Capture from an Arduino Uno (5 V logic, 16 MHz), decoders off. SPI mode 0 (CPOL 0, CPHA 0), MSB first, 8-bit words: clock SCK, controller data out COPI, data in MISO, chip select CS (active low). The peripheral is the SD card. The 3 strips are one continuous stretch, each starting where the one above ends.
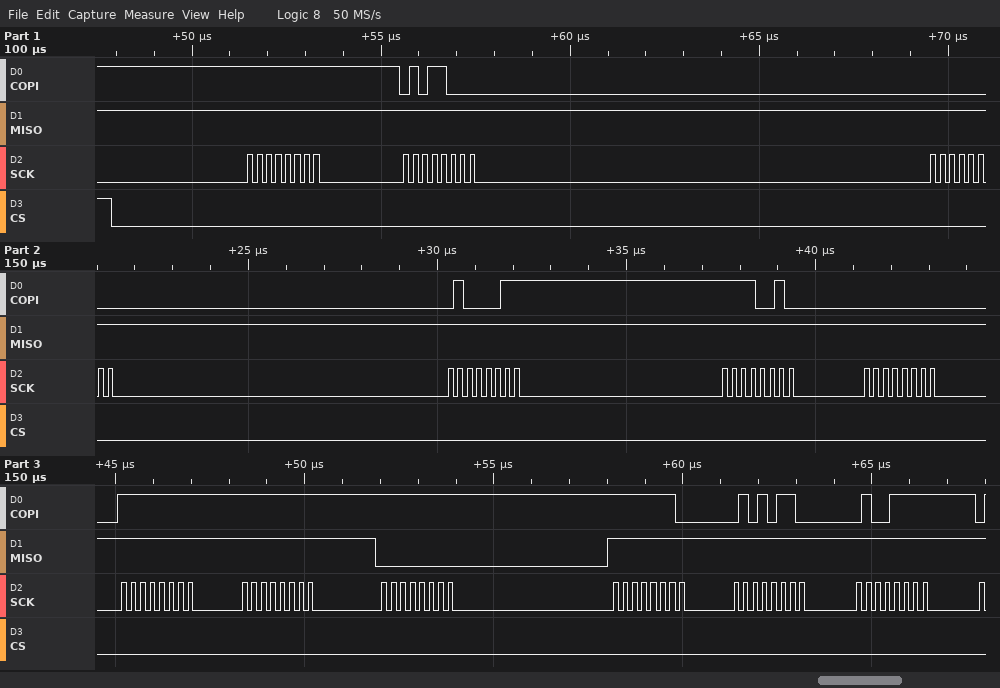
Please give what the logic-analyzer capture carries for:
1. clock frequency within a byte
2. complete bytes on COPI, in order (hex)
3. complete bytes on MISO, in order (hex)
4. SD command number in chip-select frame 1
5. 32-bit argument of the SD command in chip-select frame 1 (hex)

4 MHz
FF 58 00 43 F2 00 FF FF FF FE 56 4F
FF FF FF FF FF FF FF FF 00 FF FF FF
CMD24
0x0043F200
